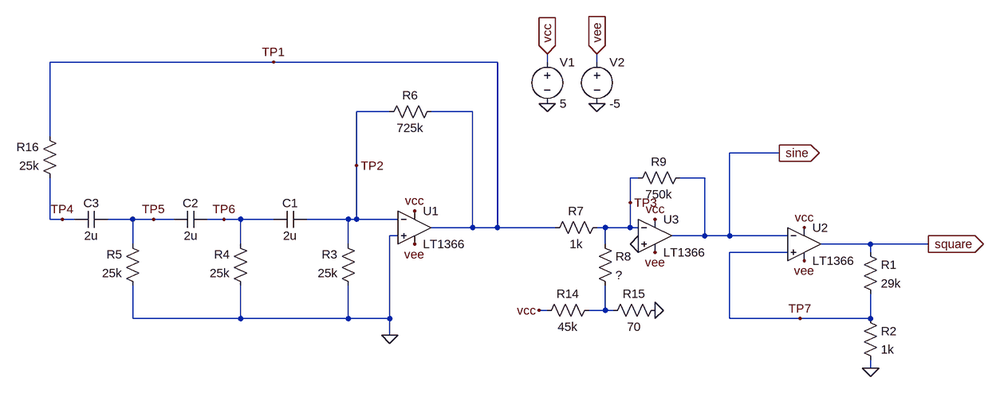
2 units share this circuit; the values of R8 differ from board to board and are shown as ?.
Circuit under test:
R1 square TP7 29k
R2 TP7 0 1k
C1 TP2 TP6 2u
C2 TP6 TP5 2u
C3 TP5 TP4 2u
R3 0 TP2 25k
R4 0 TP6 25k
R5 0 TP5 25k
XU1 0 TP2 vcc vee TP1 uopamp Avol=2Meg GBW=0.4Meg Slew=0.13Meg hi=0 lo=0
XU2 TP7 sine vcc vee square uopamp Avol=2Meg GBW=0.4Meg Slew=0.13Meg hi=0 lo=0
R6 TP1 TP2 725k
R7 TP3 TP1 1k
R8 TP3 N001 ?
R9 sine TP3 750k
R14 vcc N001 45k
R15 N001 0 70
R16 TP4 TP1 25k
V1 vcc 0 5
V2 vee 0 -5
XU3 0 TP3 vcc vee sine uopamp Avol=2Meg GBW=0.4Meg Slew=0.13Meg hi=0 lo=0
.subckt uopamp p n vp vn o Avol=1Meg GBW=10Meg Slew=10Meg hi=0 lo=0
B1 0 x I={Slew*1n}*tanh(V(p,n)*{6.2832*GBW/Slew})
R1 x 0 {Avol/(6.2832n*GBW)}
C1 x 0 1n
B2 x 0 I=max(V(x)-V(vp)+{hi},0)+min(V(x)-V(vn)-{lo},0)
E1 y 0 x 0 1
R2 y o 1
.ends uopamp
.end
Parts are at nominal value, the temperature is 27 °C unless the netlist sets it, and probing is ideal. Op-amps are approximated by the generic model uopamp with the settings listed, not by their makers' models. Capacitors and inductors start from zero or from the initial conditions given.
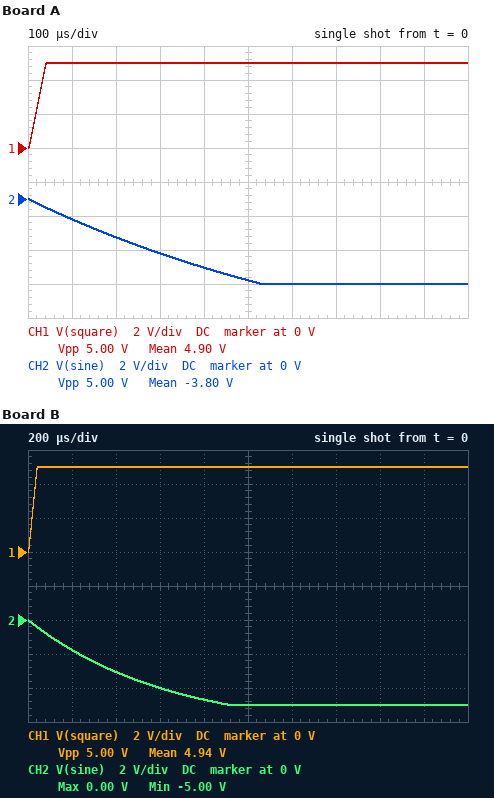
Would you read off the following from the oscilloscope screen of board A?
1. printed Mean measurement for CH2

-3.80 V
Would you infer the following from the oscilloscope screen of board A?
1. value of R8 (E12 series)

470 Ω
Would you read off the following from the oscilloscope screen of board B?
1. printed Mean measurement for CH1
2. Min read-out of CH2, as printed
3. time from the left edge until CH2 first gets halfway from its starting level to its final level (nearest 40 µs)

4.94 V
-5.00 V
320 µs
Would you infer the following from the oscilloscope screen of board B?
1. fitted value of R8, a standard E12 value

820 Ω
